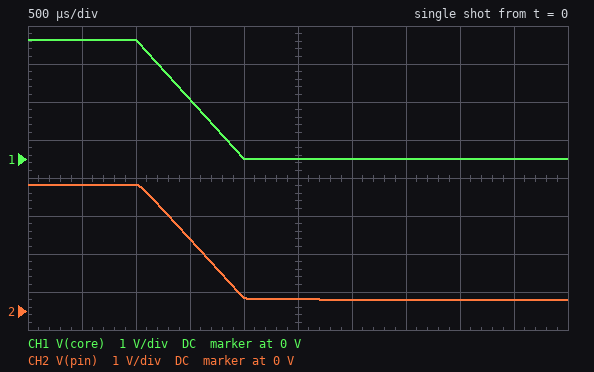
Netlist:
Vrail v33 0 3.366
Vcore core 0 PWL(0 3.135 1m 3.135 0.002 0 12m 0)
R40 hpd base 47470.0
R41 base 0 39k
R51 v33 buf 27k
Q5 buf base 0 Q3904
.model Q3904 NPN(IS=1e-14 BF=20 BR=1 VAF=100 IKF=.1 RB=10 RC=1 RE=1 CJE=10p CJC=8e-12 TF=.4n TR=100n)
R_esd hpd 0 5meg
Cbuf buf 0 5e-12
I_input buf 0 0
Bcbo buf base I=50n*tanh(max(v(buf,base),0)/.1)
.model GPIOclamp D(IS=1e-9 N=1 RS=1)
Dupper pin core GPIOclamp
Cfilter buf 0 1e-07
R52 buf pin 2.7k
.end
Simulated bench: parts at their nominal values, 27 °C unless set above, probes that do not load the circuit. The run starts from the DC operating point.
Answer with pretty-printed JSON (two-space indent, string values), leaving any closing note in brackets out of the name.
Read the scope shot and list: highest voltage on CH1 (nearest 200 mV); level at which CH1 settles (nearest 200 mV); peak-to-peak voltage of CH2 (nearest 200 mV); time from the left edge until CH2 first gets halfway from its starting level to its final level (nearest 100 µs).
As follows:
{
  "highest voltage on CH1": "3.2 V",
  "level at which CH1 settles": "0 V",
  "peak-to-peak voltage of CH2": "3.0 V",
  "time from the left edge until CH2 first gets halfway from its starting level to its final level": "1.5 ms"
}
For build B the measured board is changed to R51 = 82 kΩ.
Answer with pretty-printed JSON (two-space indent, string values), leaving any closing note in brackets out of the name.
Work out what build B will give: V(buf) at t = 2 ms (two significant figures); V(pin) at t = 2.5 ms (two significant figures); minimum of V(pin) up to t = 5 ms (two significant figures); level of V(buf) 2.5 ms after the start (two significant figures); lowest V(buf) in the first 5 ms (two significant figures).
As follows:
{
  "V(buf) at t = 2 ms": "1.2 V",
  "V(pin) at t = 2.5 ms": "290 mV",
  "minimum of V(pin) up to t = 5 ms": "270 mV",
  "level of V(buf) 2.5 ms after the start": "520 mV",
  "lowest V(buf) in the first 5 ms": "370 mV"
}
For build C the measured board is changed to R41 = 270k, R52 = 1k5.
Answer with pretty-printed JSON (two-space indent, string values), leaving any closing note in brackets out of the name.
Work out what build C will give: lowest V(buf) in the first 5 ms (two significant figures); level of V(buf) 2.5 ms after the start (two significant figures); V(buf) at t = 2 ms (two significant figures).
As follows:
{
  "lowest V(buf) in the first 5 ms": "460 mV",
  "level of V(buf) 2.5 ms after the start": "480 mV",
  "V(buf) at t = 2 ms": "910 mV"
}
